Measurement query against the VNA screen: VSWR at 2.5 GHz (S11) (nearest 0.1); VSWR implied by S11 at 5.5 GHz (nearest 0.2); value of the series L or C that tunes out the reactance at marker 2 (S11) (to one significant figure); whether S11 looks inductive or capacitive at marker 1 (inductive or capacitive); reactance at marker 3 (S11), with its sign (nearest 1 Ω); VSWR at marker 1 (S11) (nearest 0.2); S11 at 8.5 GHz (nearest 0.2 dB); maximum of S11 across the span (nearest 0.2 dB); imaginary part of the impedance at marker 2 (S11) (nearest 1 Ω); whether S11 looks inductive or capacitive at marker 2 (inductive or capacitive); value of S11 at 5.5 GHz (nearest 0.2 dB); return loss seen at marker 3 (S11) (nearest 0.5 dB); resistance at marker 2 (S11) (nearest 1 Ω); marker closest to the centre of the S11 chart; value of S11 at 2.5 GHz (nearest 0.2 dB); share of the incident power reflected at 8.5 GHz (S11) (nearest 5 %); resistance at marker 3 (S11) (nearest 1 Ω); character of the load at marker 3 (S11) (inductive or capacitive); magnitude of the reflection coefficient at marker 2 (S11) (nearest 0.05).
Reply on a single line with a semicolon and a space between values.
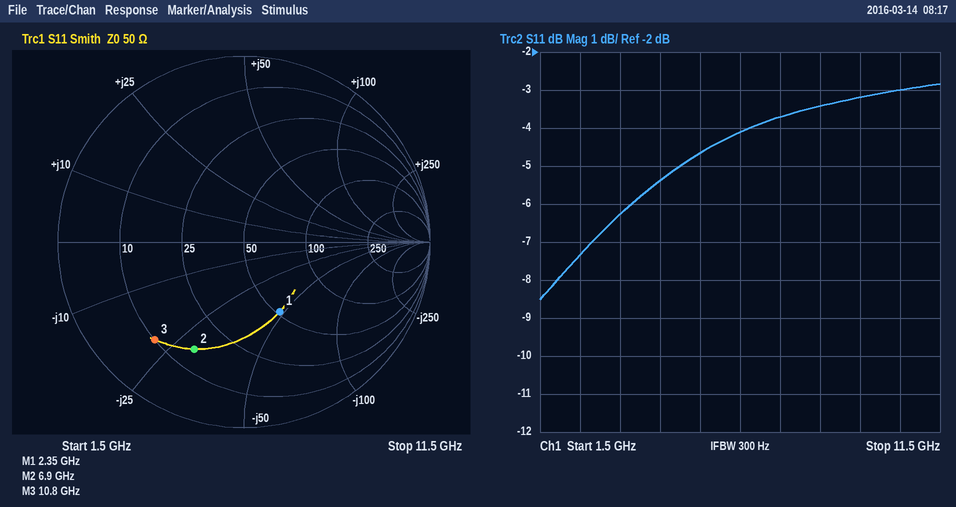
2.5; 3.8; 700 pH; capacitive; -21 Ω; 2.4; -3.4 dB; -2.8 dB; -30 Ω; capacitive; -4.6 dB; 3.0 dB; 15 Ω; marker 1; -7.4 dB; 45 %; 10 Ω; capacitive; 0.65
